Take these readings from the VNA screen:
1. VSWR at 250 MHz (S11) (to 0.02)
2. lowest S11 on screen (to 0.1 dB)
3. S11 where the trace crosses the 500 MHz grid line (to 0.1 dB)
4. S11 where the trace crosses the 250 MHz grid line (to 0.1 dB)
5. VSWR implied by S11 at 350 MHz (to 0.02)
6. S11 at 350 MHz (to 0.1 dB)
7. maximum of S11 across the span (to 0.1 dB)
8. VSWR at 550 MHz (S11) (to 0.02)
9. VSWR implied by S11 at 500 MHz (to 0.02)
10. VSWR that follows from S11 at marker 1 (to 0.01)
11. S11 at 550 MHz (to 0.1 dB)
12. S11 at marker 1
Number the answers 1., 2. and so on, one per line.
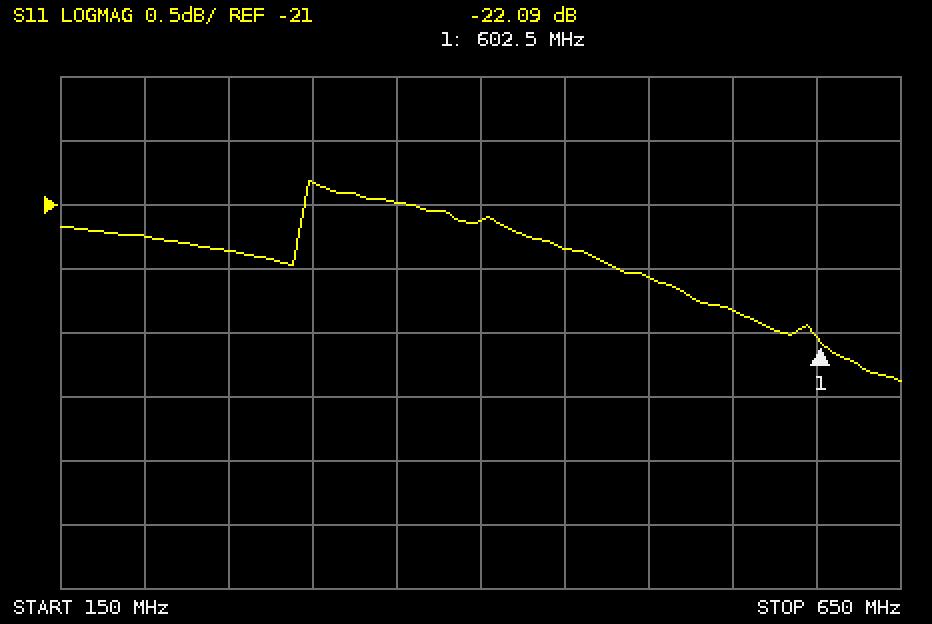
1. 1.18
2. -22.4 dB
3. -21.6 dB
4. -21.4 dB
5. 1.20
6. -21.0 dB
7. -20.8 dB
8. 1.18
9. 1.18
10. 1.17
11. -21.8 dB
12. -22.09 dB
